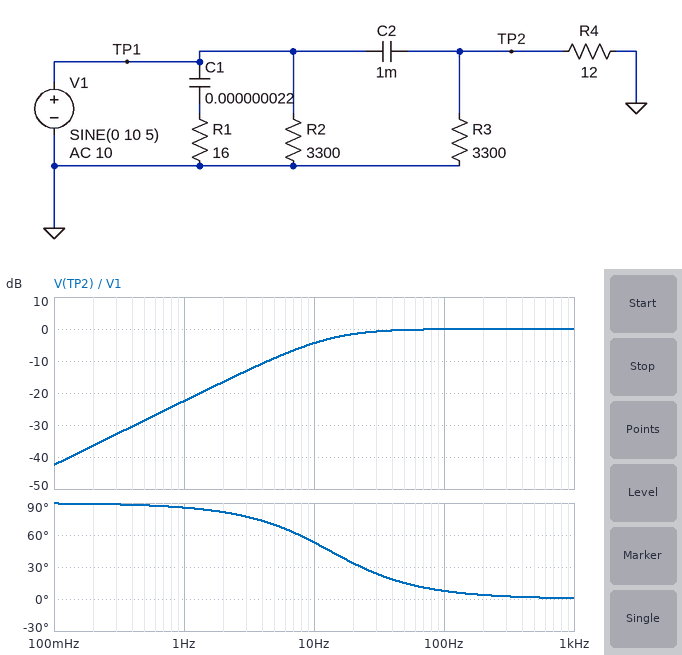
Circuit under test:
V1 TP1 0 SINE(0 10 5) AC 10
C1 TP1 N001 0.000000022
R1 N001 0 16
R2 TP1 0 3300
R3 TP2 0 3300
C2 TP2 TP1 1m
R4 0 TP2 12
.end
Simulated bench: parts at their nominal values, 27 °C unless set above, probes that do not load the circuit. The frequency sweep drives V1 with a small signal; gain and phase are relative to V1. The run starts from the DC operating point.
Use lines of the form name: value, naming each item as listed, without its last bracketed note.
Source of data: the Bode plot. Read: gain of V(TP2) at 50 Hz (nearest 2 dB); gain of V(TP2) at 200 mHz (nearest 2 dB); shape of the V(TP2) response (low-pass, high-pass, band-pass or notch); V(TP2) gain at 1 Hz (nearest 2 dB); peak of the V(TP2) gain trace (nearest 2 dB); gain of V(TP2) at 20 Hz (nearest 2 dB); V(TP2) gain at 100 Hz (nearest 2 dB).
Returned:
gain of V(TP2) at 50 Hz: 0 dB
gain of V(TP2) at 200 mHz: -36 dB
shape of the V(TP2) response: high-pass
V(TP2) gain at 1 Hz: -22 dB
peak of the V(TP2) gain trace: 0 dB
gain of V(TP2) at 20 Hz: -2 dB
V(TP2) gain at 100 Hz: 0 dB
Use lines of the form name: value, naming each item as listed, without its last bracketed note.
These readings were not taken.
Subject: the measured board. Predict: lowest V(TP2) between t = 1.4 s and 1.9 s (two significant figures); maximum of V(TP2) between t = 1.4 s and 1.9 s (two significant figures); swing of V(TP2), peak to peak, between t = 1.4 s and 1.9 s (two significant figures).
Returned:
lowest V(TP2) between t = 1.4 s and 1.9 s: -3.5 V
maximum of V(TP2) between t = 1.4 s and 1.9 s: 3.5 V
swing of V(TP2), peak to peak, between t = 1.4 s and 1.9 s: 7.0 V
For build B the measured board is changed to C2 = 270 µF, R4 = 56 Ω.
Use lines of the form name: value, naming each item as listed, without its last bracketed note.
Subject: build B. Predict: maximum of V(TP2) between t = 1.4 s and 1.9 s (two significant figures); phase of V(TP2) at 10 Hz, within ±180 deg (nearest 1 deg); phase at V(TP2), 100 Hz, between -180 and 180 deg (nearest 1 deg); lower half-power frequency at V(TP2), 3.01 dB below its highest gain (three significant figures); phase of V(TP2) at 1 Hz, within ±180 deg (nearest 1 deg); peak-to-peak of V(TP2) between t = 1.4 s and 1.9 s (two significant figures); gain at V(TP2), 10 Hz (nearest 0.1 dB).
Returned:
maximum of V(TP2) between t = 1.4 s and 1.9 s: 4.2 V
phase of V(TP2) at 10 Hz, within ±180 deg: 47 deg
phase at V(TP2), 100 Hz, between -180 and 180 deg: 6 deg
lower half-power frequency at V(TP2), 3.01 dB below its highest gain: 10.7 Hz
phase of V(TP2) at 1 Hz, within ±180 deg: 85 deg
peak-to-peak of V(TP2) between t = 1.4 s and 1.9 s: 8.5 V
gain at V(TP2), 10 Hz: -3.3 dB
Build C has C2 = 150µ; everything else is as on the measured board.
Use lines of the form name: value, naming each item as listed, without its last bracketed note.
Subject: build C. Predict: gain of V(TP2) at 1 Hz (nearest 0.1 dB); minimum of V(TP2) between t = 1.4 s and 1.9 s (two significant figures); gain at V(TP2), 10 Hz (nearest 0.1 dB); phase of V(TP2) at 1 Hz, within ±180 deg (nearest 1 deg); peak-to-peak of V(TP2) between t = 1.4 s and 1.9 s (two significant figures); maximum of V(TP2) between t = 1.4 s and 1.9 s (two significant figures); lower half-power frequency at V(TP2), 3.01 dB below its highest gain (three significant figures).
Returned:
gain of V(TP2) at 1 Hz: -39.0 dB
minimum of V(TP2) between t = 1.4 s and 1.9 s: -560 mV
gain at V(TP2), 10 Hz: -19.0 dB
phase of V(TP2) at 1 Hz, within ±180 deg: 89 deg
peak-to-peak of V(TP2) between t = 1.4 s and 1.9 s: 1.1 V
maximum of V(TP2) between t = 1.4 s and 1.9 s: 560 mV
lower half-power frequency at V(TP2), 3.01 dB below its highest gain: 88.7 Hz
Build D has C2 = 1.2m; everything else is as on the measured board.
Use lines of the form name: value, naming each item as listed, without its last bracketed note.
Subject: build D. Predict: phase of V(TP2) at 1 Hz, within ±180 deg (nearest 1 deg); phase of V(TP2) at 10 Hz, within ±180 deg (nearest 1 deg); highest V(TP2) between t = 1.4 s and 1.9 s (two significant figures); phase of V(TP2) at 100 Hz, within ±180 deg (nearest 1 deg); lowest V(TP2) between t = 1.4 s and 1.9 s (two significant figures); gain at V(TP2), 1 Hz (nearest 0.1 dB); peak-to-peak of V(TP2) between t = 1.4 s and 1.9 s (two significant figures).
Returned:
phase of V(TP2) at 1 Hz, within ±180 deg: 85 deg
phase of V(TP2) at 10 Hz, within ±180 deg: 48 deg
highest V(TP2) between t = 1.4 s and 1.9 s: 4.1 V
phase of V(TP2) at 100 Hz, within ±180 deg: 6 deg
lowest V(TP2) between t = 1.4 s and 1.9 s: -4.1 V
gain at V(TP2), 1 Hz: -20.9 dB
peak-to-peak of V(TP2) between t = 1.4 s and 1.9 s: 8.2 V
